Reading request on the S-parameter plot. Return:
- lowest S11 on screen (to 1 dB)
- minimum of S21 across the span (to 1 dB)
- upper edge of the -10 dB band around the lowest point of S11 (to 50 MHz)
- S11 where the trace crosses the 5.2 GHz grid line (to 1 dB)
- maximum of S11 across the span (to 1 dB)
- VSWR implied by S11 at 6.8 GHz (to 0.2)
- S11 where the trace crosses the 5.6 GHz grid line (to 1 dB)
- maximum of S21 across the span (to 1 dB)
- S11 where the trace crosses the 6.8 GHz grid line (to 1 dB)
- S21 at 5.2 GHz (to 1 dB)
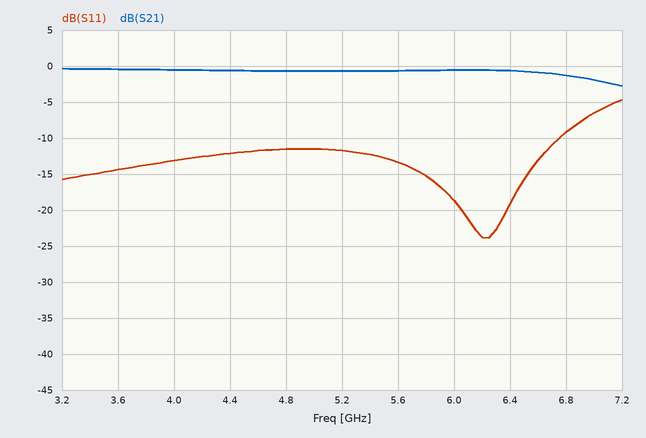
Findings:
-24 dB
-3 dB
6.75 GHz
-12 dB
-5 dB
2.0
-13 dB
0 dB
-9 dB
-1 dB
